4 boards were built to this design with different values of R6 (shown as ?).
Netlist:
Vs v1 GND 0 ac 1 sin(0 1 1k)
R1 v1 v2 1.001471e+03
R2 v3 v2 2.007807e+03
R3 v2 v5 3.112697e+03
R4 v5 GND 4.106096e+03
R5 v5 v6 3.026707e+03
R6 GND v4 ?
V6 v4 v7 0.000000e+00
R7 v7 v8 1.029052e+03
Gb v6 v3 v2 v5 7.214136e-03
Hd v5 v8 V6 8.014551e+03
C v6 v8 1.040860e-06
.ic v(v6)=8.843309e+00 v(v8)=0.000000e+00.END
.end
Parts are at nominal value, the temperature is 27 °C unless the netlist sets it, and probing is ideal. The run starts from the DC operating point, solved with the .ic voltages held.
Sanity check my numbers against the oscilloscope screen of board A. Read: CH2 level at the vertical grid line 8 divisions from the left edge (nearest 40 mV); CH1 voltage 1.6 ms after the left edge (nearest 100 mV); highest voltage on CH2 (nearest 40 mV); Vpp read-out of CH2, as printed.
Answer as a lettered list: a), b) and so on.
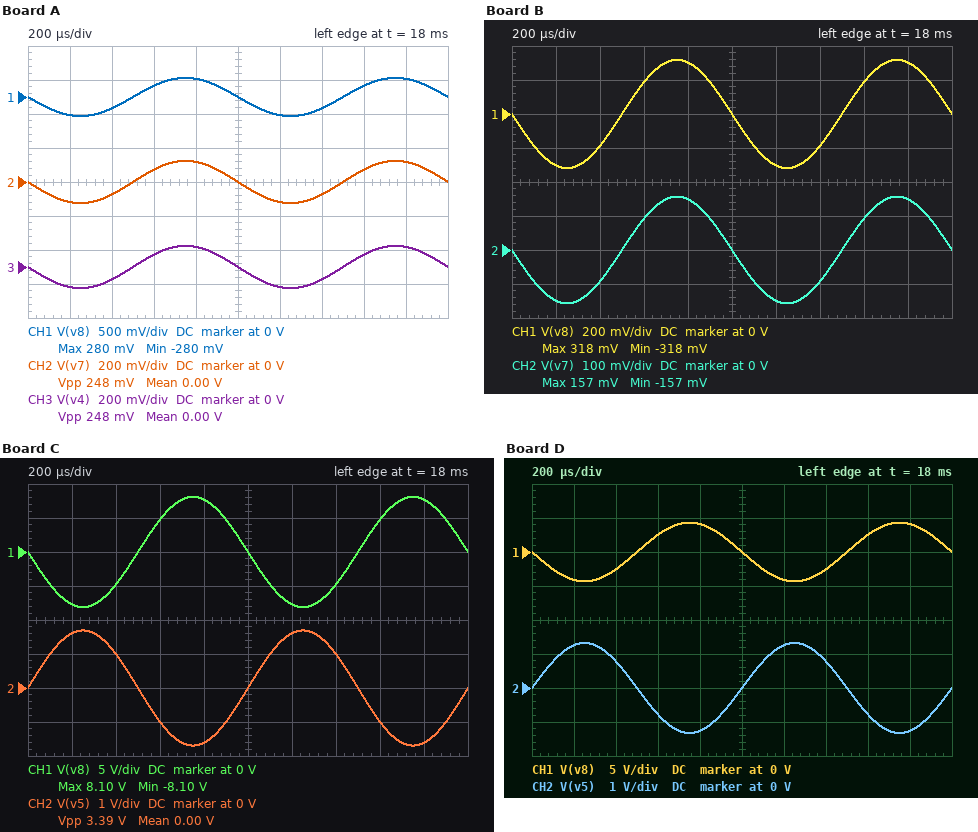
a) 80 mV
b) 200 mV
c) 120 mV
d) 248 mV
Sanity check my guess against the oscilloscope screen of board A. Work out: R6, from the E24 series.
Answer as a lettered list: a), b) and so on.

a) 820 Ω
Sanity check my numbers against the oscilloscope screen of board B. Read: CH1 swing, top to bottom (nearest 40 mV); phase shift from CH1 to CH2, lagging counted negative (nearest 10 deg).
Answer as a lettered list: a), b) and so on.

a) 640 mV
b) 0 deg
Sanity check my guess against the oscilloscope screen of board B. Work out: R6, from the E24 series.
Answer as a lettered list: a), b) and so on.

a) 1 kΩ
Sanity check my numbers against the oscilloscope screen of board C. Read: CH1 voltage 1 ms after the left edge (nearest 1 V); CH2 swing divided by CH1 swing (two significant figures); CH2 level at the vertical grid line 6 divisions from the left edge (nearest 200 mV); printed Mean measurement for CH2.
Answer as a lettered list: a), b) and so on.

a) 0 V
b) 0.21
c) 1.6 V
d) 0.00 V
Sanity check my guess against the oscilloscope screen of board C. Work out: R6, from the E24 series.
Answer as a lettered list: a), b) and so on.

a) 5.6 kΩ
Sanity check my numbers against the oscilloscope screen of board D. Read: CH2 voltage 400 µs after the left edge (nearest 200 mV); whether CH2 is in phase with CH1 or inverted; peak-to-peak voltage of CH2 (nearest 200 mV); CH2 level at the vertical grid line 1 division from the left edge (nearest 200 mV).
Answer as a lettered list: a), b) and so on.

a) 800 mV
b) inverted
c) 2.6 V
d) 1.2 V
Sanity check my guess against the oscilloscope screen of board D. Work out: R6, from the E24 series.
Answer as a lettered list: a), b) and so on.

a) 5.1 kΩ
